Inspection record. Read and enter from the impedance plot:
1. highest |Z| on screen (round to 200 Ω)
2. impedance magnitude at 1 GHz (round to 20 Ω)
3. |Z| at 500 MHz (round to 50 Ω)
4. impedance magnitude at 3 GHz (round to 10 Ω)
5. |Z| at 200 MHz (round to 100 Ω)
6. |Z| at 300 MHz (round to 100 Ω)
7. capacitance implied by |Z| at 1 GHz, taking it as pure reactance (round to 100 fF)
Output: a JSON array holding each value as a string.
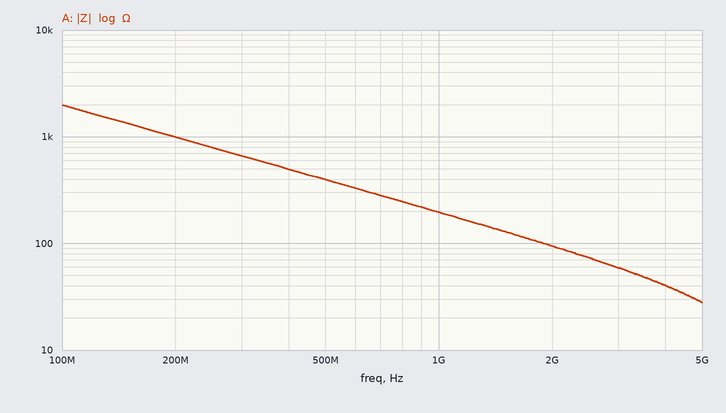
["2.0 kΩ", "200 Ω", "400 Ω", "60 Ω", "1.0 kΩ", "700 Ω", "800 fF"]
